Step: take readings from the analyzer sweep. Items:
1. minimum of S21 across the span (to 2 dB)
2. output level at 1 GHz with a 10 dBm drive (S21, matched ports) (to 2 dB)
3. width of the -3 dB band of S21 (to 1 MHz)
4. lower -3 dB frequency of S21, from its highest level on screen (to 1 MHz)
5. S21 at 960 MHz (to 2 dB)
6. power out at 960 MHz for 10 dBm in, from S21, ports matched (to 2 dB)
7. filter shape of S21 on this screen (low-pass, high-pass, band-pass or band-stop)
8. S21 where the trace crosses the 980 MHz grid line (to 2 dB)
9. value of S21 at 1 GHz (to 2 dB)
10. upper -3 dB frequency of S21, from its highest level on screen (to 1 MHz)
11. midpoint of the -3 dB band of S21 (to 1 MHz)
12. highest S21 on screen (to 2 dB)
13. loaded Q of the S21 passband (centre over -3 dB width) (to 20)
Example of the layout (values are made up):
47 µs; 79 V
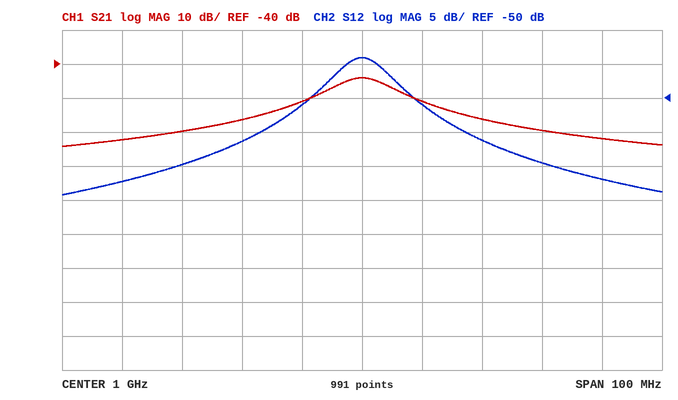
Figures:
-64 dB; -34 dBm; 10 MHz; 995 MHz; -62 dB; -52 dBm; band-pass; -56 dB; -44 dB; 1.005 GHz; 1.000 GHz; -44 dB; 100
